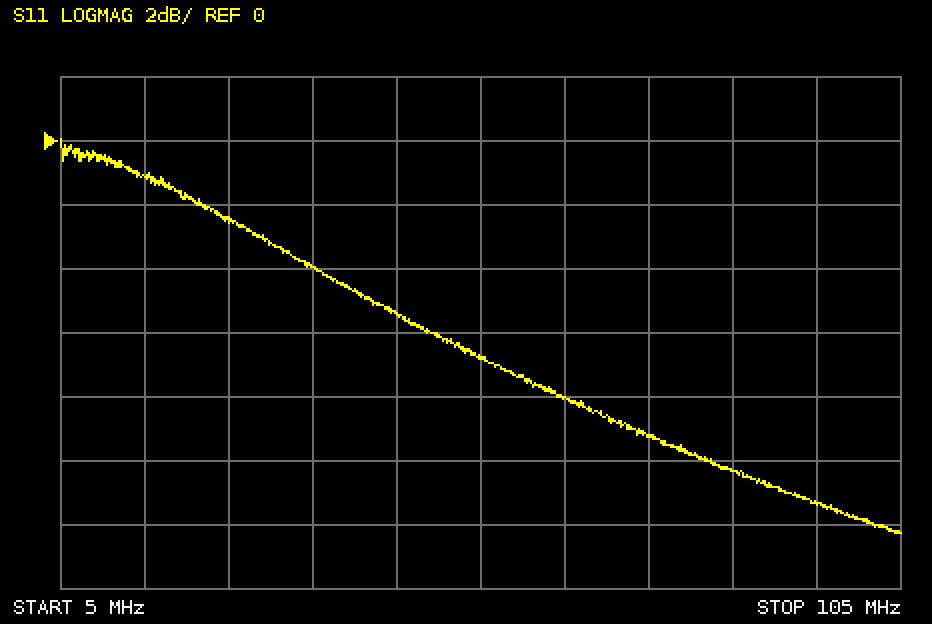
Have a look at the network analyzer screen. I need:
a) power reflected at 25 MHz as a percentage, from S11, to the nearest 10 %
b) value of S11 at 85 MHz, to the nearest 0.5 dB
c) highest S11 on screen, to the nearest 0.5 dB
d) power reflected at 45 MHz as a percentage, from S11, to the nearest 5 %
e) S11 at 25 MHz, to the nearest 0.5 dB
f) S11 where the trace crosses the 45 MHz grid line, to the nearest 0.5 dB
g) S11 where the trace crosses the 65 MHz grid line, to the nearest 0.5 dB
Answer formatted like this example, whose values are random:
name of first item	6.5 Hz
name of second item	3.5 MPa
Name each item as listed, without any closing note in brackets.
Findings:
power reflected at 25 MHz as a percentage, from S11, to the nearest 10 %	60 %
value of S11 at 85 MHz, to the nearest 0.5 dB	-10.5 dB
highest S11 on screen, to the nearest 0.5 dB	0.0 dB
power reflected at 45 MHz as a percentage, from S11, to the nearest 5 %	30 %
S11 at 25 MHz, to the nearest 0.5 dB	-2.5 dB
S11 where the trace crosses the 45 MHz grid line, to the nearest 0.5 dB	-5.5 dB
S11 where the trace crosses the 65 MHz grid line, to the nearest 0.5 dB	-8.0 dB
